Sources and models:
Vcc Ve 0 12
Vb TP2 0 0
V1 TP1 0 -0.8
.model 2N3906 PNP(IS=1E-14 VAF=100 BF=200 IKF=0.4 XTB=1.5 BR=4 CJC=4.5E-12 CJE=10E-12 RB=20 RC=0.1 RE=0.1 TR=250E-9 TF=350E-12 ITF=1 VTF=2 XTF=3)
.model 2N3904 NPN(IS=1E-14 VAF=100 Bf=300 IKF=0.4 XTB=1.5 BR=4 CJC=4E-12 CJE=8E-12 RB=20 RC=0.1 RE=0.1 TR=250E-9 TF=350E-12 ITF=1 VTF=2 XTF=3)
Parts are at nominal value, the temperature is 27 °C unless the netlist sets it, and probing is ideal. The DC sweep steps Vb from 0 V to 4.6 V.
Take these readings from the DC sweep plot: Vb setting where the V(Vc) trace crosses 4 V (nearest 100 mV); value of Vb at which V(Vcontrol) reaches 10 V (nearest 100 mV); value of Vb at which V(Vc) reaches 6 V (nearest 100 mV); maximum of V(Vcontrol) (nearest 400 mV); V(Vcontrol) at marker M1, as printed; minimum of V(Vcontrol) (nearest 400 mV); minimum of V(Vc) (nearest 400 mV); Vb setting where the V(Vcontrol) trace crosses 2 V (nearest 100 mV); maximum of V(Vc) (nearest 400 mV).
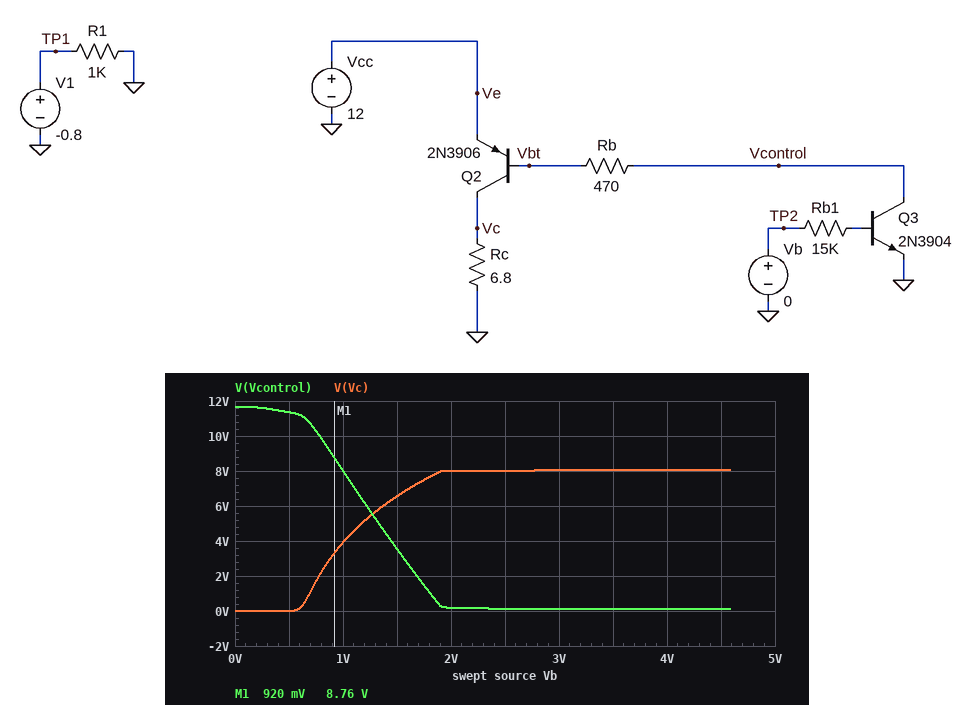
1.0 V
800 mV
1.4 V
11.6 V
8.76 V
0 V
0 V
1.7 V
8.0 V
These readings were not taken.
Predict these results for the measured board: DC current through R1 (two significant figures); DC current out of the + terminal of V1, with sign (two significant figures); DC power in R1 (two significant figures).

800 µA
-800 µA
640 µW
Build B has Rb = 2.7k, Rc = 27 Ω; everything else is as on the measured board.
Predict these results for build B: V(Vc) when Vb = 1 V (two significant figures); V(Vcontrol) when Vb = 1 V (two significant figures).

11 V
130 mV
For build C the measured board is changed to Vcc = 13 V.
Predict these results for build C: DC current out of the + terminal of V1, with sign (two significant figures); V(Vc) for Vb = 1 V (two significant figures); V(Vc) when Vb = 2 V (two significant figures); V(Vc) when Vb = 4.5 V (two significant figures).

-800 µA
4.0 V
8.4 V
8.5 V
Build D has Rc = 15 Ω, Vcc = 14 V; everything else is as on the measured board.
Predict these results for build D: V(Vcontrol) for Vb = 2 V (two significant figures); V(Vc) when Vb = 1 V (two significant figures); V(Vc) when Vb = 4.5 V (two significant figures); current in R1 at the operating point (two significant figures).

1.3 V
8.5 V
14 V
800 µA
